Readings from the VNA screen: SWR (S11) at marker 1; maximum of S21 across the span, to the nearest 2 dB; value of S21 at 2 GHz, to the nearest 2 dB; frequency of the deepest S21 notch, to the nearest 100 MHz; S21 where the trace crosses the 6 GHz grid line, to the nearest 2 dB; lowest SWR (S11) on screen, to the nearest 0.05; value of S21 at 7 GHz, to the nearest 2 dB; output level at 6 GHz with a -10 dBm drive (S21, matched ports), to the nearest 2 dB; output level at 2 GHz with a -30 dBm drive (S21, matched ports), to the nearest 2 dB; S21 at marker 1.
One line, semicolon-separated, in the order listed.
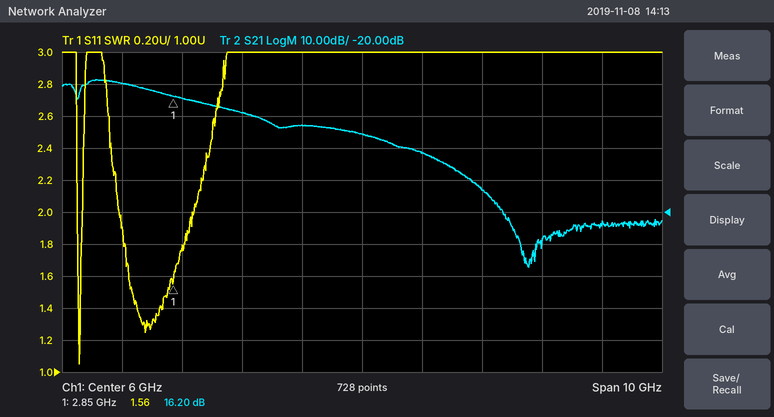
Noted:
1.56; 22 dB; 20 dB; 8.8 GHz; 4 dB; 1.05; -2 dB; -6 dBm; -10 dBm; 16.20 dB
